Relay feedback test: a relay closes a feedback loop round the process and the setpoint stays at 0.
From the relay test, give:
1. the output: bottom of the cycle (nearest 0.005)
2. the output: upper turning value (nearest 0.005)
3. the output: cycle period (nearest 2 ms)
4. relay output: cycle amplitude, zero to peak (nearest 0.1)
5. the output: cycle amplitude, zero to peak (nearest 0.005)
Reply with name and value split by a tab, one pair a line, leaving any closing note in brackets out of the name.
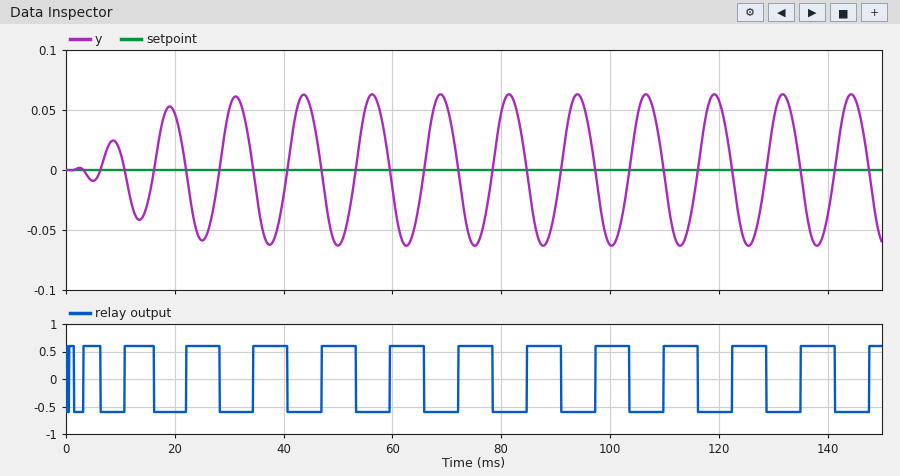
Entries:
the output: bottom of the cycle	-0.065
the output: upper turning value	0.065
the output: cycle period	12 ms
relay output: cycle amplitude, zero to peak	0.6
the output: cycle amplitude, zero to peak	0.065
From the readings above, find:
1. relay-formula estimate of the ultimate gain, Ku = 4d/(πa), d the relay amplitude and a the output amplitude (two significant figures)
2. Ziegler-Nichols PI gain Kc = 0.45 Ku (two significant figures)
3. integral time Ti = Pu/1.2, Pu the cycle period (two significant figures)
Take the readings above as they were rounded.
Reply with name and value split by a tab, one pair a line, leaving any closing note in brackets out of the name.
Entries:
relay-formula estimate of the ultimate gain, Ku = 4d/(πa), d the relay amplitude and a the output amplitude	12
Ziegler-Nichols PI gain Kc = 0.45 Ku	5.4
integral time Ti = Pu/1.2, Pu the cycle period	10 ms
